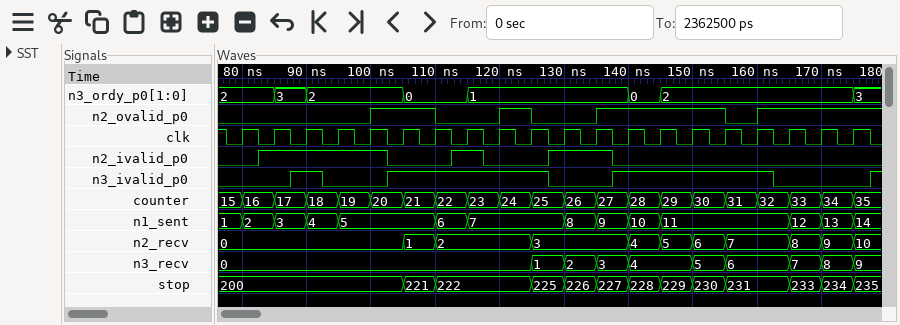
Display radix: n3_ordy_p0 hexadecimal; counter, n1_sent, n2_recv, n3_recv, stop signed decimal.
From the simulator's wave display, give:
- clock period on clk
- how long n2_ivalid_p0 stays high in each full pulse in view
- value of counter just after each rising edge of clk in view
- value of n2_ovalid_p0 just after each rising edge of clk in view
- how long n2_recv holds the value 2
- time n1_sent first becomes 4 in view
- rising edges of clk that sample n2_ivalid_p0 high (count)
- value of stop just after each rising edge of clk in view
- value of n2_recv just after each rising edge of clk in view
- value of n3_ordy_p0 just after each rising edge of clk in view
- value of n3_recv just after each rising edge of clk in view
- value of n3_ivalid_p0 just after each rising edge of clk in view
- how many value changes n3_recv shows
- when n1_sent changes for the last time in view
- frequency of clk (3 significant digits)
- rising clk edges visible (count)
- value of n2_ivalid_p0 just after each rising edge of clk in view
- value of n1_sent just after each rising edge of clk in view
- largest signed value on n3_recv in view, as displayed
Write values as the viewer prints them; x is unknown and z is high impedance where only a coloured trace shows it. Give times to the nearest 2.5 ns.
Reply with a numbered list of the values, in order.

1. 5 ns
2. 20 ns, 5 ns, 10 ns
3. 16, 17, 18, 19, 20, 21, 22, 23, 24, 25, 26, 27, 28, 29, 30, 31, 32, 33, 34, 35
4. 0 0 0 0 1 1 0 0 1 0 0 1 1 1 1 0 1 1 1 1
5. 15 ns
6. 90 ns
7. 7
8. 200, 200, 200, 200, 200, 221, 222, 222, 222, 225, 226, 227, 228, 229, 230, 231, 231, 233, 234, 235
9. 0, 0, 0, 0, 0, 1, 2, 2, 2, 3, 3, 3, 4, 5, 6, 7, 7, 8, 9, 10
10. 2, 3, 2, 2, 2, 0, 0, 1, 1, 1, 1, 1, 0, 2, 2, 2, 2, 2, 2, 3
11. 0, 0, 0, 0, 0, 0, 0, 0, 0, 1, 2, 3, 4, 4, 5, 6, 6, 7, 8, 9
12. 0 0 1 0 0 1 1 1 1 1 0 0 1 1 1 1 1 0 0 0
13. 9
14. 175 ns
15. 200 MHz
16. 20
17. 0 1 1 1 1 0 0 1 0 0 1 1 0 0 0 0 0 0 0 0
18. 2, 3, 4, 5, 5, 5, 6, 7, 7, 7, 8, 9, 10, 11, 11, 11, 11, 12, 13, 14
19. 9
